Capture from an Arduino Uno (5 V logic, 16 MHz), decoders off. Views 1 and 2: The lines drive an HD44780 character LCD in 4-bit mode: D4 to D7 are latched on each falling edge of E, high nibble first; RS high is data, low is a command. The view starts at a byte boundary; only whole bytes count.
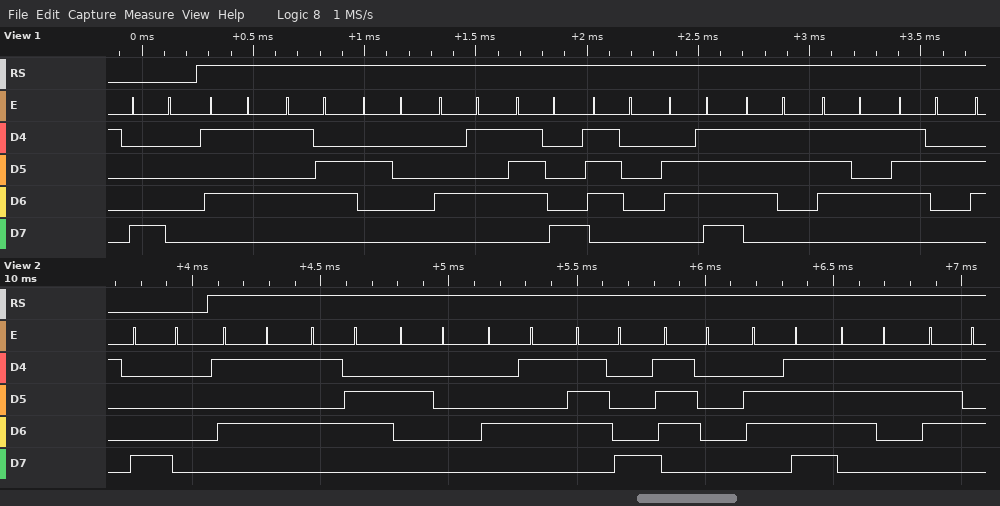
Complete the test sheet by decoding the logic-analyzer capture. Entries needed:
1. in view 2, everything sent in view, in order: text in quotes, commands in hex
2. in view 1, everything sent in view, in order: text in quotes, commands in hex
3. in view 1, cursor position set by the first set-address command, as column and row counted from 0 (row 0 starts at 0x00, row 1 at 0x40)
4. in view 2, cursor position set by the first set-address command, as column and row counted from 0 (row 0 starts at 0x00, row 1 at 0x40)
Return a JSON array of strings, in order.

["0x80 \"UV Exposu\"", "0x80 \"UV Exposur\"", "column 0, row 0", "column 0, row 0"]
